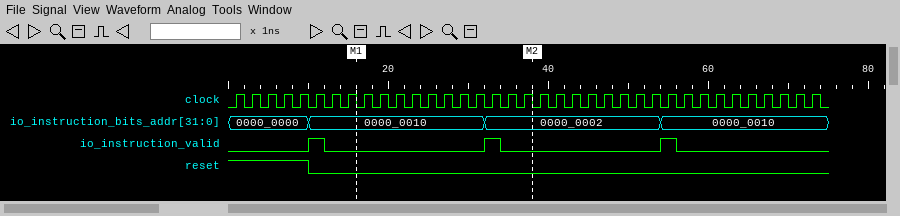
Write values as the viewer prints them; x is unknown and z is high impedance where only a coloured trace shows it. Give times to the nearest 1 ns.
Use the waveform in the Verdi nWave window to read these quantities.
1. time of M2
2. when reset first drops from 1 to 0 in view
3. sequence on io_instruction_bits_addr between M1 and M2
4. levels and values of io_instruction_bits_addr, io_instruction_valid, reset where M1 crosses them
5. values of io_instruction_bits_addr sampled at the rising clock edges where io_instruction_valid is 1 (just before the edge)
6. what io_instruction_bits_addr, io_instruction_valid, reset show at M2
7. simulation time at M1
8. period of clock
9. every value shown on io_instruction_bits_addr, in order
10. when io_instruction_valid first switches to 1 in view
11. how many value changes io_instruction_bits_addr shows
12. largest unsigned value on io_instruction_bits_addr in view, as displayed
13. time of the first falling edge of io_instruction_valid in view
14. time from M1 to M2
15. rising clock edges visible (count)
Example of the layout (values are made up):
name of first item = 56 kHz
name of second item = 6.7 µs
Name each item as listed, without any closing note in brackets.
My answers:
time of M2 = 38 ns
when reset first drops from 1 to 0 in view = 10 ns
sequence on io_instruction_bits_addr between M1 and M2 = 0000_0010, 0000_0002
levels and values of io_instruction_bits_addr, io_instruction_valid, reset where M1 crosses them = io_instruction_bits_addr=0000_0010, io_instruction_valid=0, reset=0
values of io_instruction_bits_addr sampled at the rising clock edges where io_instruction_valid is 1 = 0000_0010, 0000_0002, 0000_0010
what io_instruction_bits_addr, io_instruction_valid, reset show at M2 = io_instruction_bits_addr=0000_0002, io_instruction_valid=0, reset=0
simulation time at M1 = 16 ns
period of clock = 2 ns
every value shown on io_instruction_bits_addr, in order = 0000_0000, 0000_0010, 0000_0002, 0000_0010
when io_instruction_valid first switches to 1 in view = 10 ns
how many value changes io_instruction_bits_addr shows = 3
largest unsigned value on io_instruction_bits_addr in view, as displayed = 0000_0010
time of the first falling edge of io_instruction_valid in view = 12 ns
time from M1 to M2 = 22 ns
rising clock edges visible = 37
